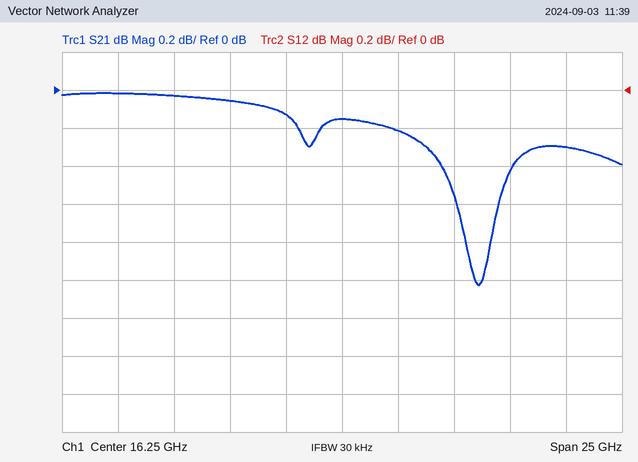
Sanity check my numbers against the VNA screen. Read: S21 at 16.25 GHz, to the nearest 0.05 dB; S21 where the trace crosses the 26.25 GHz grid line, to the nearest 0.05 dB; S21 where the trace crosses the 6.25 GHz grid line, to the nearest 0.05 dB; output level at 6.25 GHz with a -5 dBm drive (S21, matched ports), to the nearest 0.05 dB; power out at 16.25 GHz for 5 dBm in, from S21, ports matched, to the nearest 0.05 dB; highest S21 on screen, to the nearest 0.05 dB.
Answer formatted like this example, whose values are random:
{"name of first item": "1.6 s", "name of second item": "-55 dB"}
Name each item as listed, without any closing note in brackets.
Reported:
{"S21 at 16.25 GHz, to the nearest 0.05 dB": "-0.15 dB", "S21 where the trace crosses the 26.25 GHz grid line, to the nearest 0.05 dB": "-0.30 dB", "S21 where the trace crosses the 6.25 GHz grid line, to the nearest 0.05 dB": "0.00 dB", "output level at 6.25 GHz with a -5 dBm drive (S21, matched ports), to the nearest 0.05 dB": "-5.00 dBm", "power out at 16.25 GHz for 5 dBm in, from S21, ports matched, to the nearest 0.05 dB": "4.85 dBm", "highest S21 on screen, to the nearest 0.05 dB": "0.00 dB"}
